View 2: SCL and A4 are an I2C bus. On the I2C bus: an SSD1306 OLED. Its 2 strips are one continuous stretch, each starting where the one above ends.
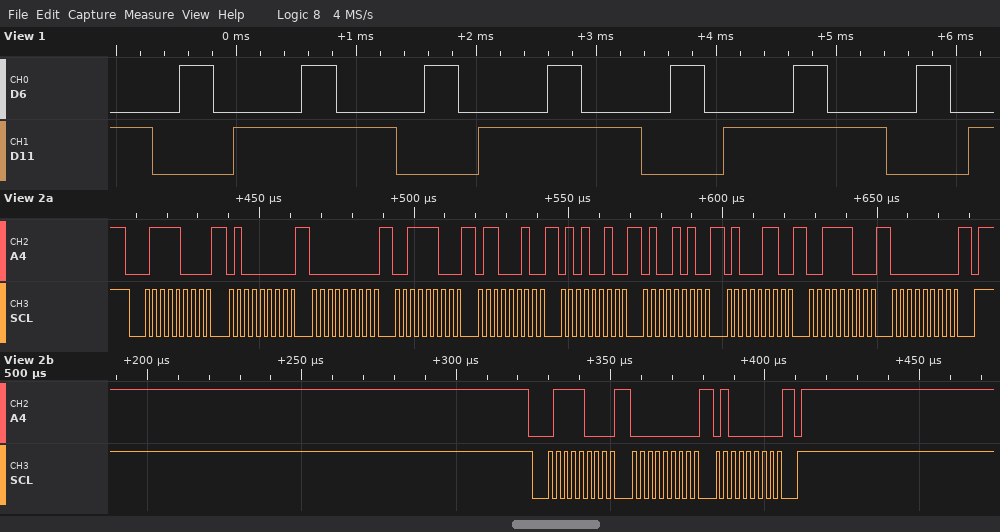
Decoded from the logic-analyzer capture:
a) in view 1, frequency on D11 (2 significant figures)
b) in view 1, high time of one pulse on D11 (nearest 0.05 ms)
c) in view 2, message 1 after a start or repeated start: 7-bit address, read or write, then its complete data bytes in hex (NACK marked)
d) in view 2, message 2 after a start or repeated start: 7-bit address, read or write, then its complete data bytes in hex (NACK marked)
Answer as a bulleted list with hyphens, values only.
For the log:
- 490 Hz
- 1.35 ms
- 0x3C write: 40 00 3C 62 52 4A 46 3C 00
- 0x3C write: 00 40
